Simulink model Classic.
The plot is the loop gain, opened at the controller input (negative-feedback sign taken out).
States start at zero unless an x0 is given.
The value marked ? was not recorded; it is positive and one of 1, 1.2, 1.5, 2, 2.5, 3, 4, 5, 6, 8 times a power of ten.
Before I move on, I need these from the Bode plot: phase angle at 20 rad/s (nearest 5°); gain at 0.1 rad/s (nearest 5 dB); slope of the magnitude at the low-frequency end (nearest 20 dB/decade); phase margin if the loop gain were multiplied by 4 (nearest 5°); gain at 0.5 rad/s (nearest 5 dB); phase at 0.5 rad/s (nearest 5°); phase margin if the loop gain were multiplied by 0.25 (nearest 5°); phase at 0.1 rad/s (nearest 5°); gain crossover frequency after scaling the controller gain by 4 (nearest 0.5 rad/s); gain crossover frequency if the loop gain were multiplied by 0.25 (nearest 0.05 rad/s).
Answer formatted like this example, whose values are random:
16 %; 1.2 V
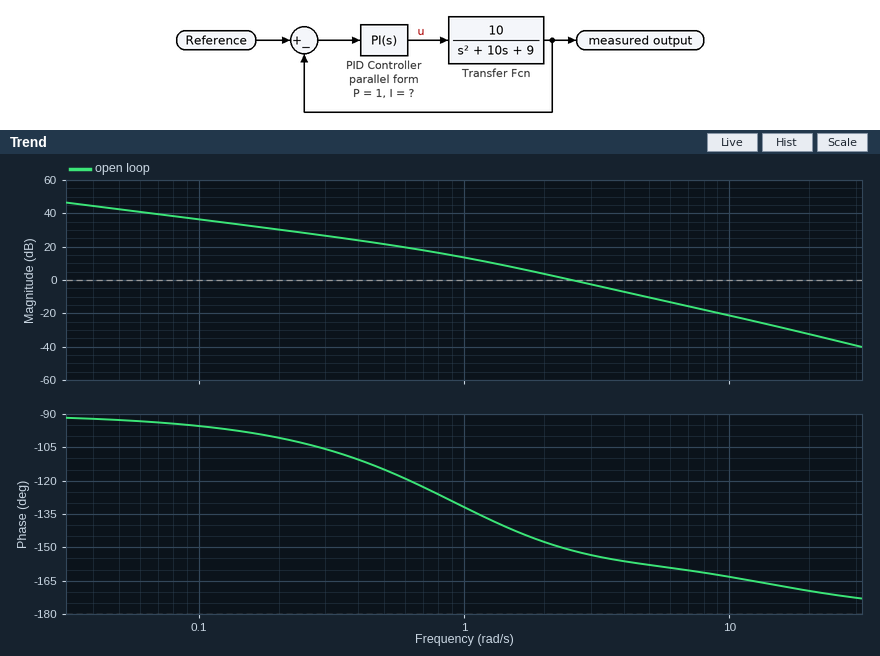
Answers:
-170°; 35 dB; -20 dB/decade; 20°; 20 dB; -115°; 45°; -95°; 5.5 rad/s; 1.10 rad/s
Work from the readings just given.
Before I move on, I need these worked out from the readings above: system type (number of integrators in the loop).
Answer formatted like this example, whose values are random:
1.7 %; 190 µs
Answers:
1
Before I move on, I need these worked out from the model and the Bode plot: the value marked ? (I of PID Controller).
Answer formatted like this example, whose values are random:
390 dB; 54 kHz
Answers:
6
